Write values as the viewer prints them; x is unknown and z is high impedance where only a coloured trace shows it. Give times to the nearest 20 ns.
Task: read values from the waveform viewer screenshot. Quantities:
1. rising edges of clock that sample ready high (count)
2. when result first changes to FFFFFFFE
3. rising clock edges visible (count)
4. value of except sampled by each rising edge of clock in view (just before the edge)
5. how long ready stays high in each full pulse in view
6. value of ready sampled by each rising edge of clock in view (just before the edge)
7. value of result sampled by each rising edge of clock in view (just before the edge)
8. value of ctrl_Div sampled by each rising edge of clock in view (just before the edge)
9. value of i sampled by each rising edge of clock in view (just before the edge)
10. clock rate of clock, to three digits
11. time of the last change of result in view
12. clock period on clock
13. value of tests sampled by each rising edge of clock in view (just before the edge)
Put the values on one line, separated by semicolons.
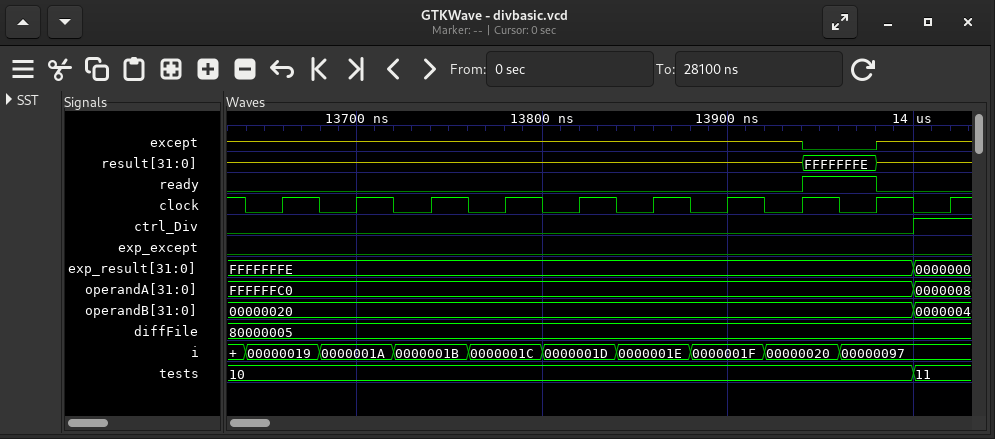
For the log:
1; 13940 ns; 10; z z z z z z z z 0 z; 40 ns; 0 0 0 0 0 0 0 0 1 0; z, z, z, z, z, z, z, z, FFFFFFFE, z; 0 0 0 0 0 0 0 0 0 1; 00000019, 0000001A, 0000001B, 0000001C, 0000001D, 0000001E, 0000001F, 00000020, 00000097, 00000097; 25.0 MHz; 13980 ns; 40 ns; 10, 10, 10, 10, 10, 10, 10, 10, 10, 11
